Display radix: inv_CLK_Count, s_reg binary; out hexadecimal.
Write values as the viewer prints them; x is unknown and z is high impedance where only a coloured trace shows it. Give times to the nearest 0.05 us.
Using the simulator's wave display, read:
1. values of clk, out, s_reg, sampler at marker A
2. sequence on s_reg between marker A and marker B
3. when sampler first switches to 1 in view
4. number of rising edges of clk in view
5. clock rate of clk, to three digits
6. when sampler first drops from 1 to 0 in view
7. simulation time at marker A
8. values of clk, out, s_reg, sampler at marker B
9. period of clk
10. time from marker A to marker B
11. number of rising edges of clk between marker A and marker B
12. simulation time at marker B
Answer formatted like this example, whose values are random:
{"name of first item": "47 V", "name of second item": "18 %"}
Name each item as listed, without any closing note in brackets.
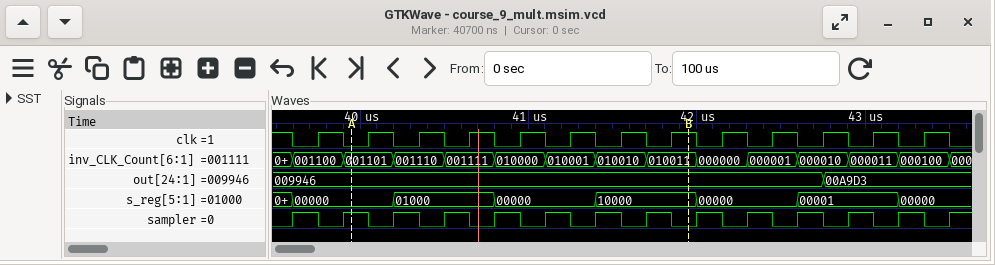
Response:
{"values of clk, out, s_reg, sampler at marker A": "clk=0, out=009946, s_reg=00000, sampler=1", "sequence on s_reg between marker A and marker B": "00000, 01000, 00000, 10000", "when sampler first switches to 1 in view": "39.6 us", "number of rising edges of clk in view": "13", "clock rate of clk, to three digits": "3.33 MHz", "when sampler first drops from 1 to 0 in view": "39.75 us", "simulation time at marker A": "39.95 us", "values of clk, out, s_reg, sampler at marker B": "clk=1, out=009946, s_reg=10000, sampler=0", "period of clk": "0.3 us", "time from marker A to marker B": "2 us", "number of rising edges of clk between marker A and marker B": "7", "simulation time at marker B": "41.95 us"}
